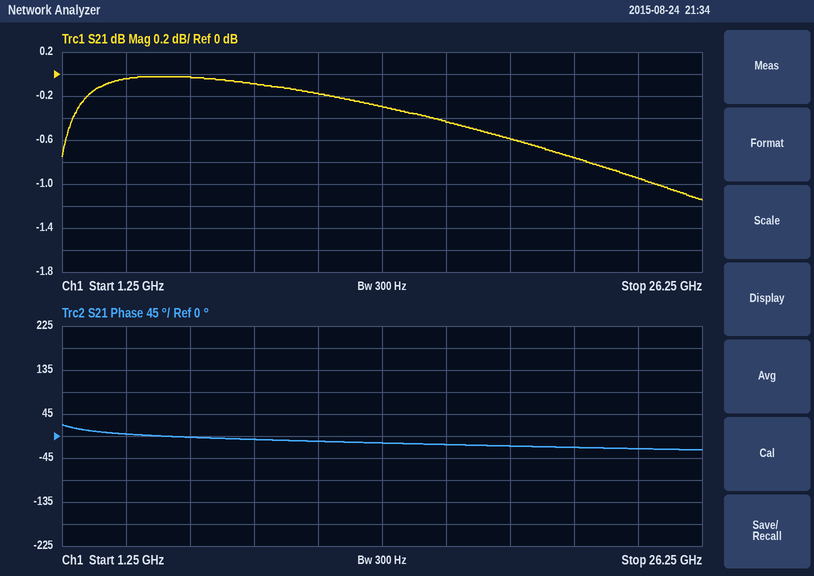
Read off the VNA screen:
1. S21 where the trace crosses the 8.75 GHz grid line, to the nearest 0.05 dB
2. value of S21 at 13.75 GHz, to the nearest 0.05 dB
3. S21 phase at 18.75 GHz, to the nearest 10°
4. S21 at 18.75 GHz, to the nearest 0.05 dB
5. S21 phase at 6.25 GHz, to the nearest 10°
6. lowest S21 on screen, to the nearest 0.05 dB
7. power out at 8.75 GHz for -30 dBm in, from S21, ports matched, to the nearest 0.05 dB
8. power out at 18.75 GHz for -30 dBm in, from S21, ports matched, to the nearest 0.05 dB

-0.10 dB
-0.30 dB
-20°
-0.60 dB
0°
-1.15 dB
-30.10 dBm
-30.60 dBm
